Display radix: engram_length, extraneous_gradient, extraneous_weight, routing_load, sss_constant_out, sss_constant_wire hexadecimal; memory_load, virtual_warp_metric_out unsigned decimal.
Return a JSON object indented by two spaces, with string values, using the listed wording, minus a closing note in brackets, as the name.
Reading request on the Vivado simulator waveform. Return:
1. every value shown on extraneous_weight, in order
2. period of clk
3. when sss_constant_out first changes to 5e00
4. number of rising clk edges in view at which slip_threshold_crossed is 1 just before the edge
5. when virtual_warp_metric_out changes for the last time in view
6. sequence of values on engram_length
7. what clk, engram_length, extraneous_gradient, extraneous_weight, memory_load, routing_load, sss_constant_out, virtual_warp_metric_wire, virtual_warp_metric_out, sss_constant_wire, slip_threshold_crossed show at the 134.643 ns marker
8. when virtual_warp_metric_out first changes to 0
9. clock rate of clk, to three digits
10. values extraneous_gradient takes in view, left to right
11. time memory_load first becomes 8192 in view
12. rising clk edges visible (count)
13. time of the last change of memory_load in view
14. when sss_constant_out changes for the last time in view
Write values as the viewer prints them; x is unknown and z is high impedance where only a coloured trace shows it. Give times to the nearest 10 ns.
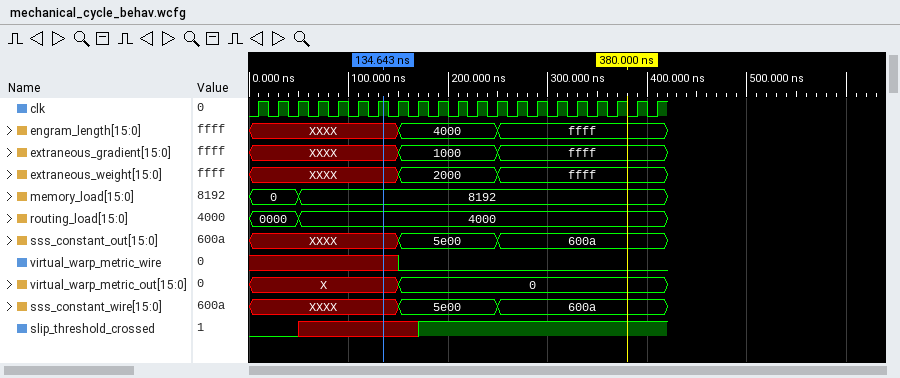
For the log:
{
  "every value shown on extraneous_weight, in order": "XXXX, 2000, ffff",
  "period of clk": "20 ns",
  "when sss_constant_out first changes to 5e00": "150 ns",
  "number of rising clk edges in view at which slip_threshold_crossed is 1 just before the edge": "12",
  "when virtual_warp_metric_out changes for the last time in view": "150 ns",
  "sequence of values on engram_length": "XXXX, 4000, ffff",
  "what clk, engram_length, extraneous_gradient, extraneous_weight, memory_load, routing_load, sss_constant_out, virtual_warp_metric_wire, virtual_warp_metric_out, sss_constant_wire, slip_threshold_crossed show at the 134.643 ns marker": "clk=1, engram_length=XXXX, extraneous_gradient=XXXX, extraneous_weight=XXXX, memory_load=8192, routing_load=4000, sss_constant_out=XXXX, virtual_warp_metric_wire=x, virtual_warp_metric_out=X, sss_constant_wire=XXXX, slip_threshold_crossed=x",
  "when virtual_warp_metric_out first changes to 0": "150 ns",
  "clock rate of clk, to three digits": "50.0 MHz",
  "values extraneous_gradient takes in view, left to right": "XXXX, 1000, ffff",
  "time memory_load first becomes 8192 in view": "50 ns",
  "rising clk edges visible": "21",
  "time of the last change of memory_load in view": "50 ns",
  "when sss_constant_out changes for the last time in view": "250 ns"
}
